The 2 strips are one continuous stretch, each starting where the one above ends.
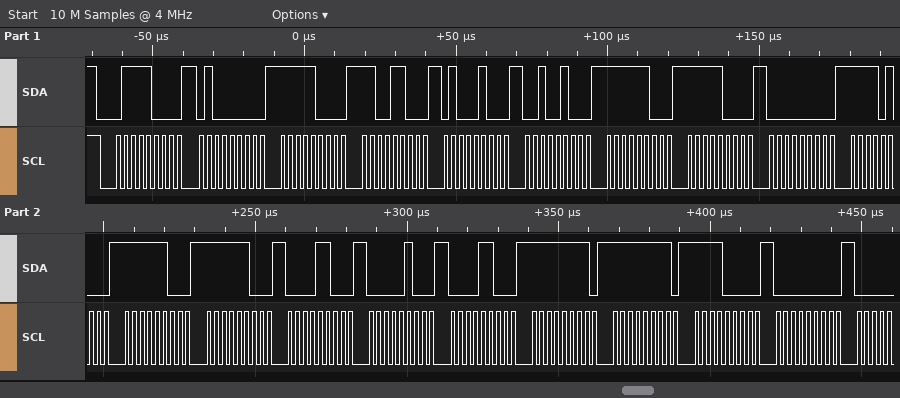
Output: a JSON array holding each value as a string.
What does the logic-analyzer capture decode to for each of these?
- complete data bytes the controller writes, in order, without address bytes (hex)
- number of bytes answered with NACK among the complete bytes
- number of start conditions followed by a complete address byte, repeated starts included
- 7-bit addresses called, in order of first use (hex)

["40 F8 CC 44 24 FC F8 00 F4 FC FC 0C 04 0C FF FF F0 00", "0", "1", "0x3C"]
